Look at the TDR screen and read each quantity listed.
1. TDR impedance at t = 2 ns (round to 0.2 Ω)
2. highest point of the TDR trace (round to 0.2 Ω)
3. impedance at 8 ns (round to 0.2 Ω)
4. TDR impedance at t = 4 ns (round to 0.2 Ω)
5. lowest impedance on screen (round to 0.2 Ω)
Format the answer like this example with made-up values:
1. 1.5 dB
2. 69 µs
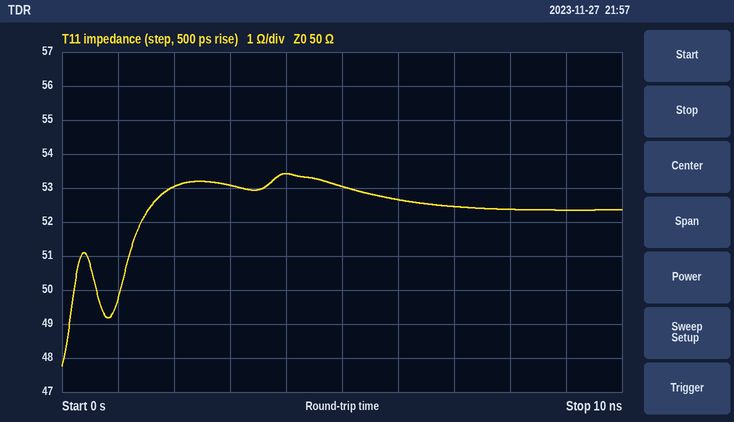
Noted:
1. 53.0 Ω
2. 53.4 Ω
3. 52.4 Ω
4. 53.4 Ω
5. 47.8 Ω
